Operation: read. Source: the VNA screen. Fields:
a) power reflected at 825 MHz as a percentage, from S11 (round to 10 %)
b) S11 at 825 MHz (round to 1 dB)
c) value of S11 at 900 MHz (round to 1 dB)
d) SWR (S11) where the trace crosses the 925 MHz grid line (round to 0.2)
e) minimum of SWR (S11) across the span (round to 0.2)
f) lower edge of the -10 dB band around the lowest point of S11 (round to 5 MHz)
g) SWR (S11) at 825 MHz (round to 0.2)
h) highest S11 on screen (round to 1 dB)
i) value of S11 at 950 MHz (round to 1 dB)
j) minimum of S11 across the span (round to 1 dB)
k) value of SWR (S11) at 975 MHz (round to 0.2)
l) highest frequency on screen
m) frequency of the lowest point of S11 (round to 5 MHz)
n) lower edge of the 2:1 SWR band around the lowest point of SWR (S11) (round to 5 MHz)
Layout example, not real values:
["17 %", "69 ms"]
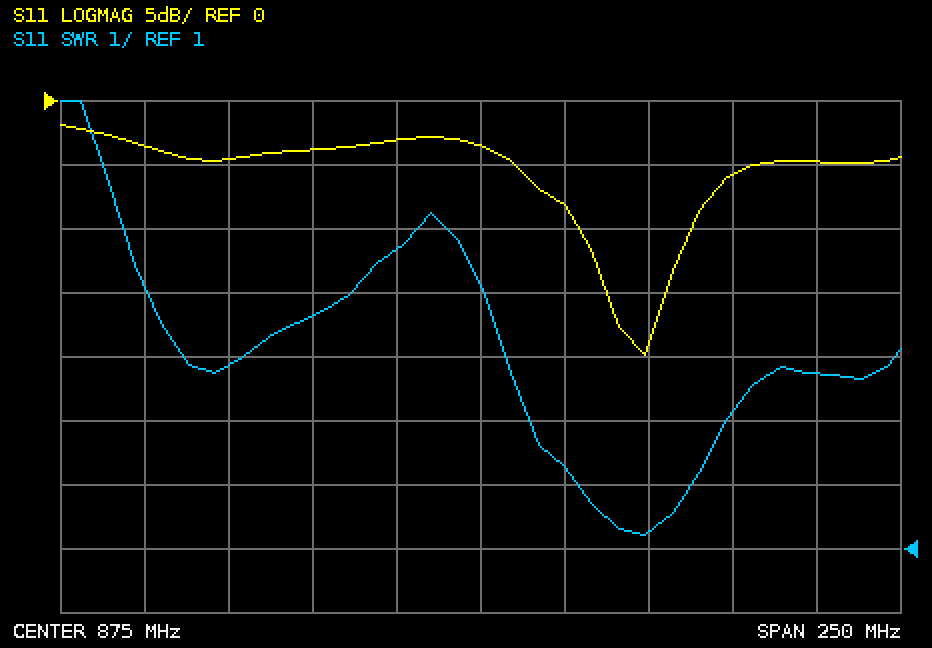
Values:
["40 %", "-4 dB", "-8 dB", "1.2", "1.2", "905 MHz", "4.6", "-2 dB", "-6 dB", "-20 dB", "3.8", "1 GHz", "925 MHz", "905 MHz"]
